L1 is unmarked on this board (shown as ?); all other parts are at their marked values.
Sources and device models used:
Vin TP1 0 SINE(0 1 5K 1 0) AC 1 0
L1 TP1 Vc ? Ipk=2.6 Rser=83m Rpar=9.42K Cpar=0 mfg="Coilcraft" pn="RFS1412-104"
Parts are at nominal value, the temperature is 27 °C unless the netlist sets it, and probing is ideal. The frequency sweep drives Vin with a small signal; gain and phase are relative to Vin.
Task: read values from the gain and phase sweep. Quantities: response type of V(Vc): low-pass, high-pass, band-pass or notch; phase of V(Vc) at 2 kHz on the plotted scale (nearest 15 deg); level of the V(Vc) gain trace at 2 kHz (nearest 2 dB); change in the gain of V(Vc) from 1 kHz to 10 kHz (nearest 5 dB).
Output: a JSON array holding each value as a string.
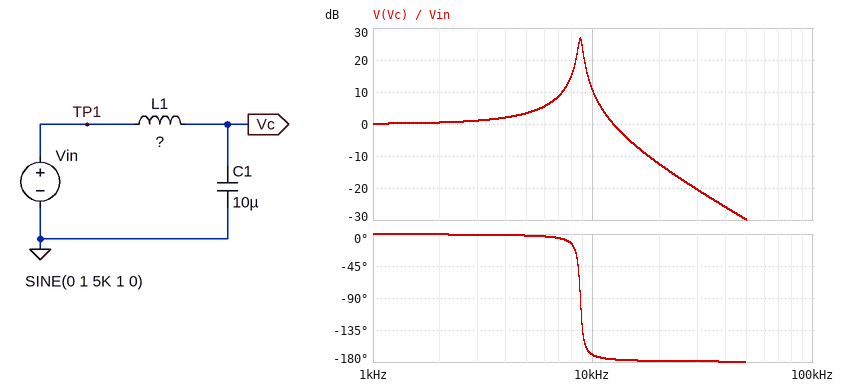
["low-pass", "0 deg", "0 dB", "10 dB"]
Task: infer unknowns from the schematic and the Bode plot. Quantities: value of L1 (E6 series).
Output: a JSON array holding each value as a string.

["33 µH"]
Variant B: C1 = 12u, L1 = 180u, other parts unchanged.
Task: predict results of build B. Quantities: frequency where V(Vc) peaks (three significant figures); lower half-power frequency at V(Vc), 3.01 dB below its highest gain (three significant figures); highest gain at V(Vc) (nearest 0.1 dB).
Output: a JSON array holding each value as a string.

["3.42 kHz", "3.39 kHz", "33.2 dB"]
